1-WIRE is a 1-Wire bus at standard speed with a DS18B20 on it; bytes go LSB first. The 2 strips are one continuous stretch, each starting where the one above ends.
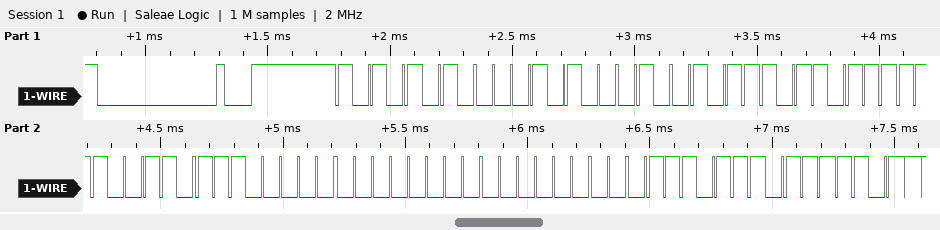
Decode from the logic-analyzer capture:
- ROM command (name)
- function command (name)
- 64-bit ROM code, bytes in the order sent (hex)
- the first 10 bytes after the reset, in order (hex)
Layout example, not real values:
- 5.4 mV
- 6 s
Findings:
- Match ROM
- Read Scratchpad
- 28 D2 ED 67 07 00 00 EE
- 55 28 D2 ED 67 07 00 00 EE BE
